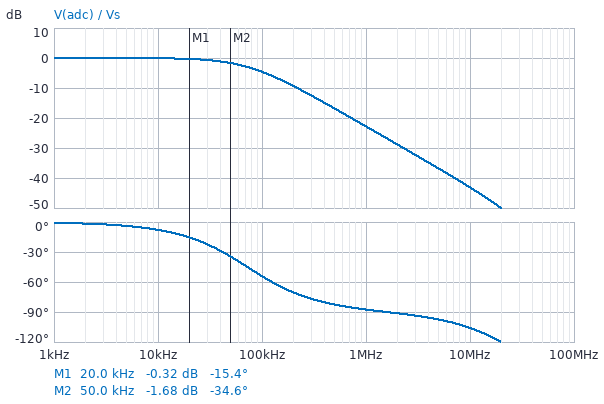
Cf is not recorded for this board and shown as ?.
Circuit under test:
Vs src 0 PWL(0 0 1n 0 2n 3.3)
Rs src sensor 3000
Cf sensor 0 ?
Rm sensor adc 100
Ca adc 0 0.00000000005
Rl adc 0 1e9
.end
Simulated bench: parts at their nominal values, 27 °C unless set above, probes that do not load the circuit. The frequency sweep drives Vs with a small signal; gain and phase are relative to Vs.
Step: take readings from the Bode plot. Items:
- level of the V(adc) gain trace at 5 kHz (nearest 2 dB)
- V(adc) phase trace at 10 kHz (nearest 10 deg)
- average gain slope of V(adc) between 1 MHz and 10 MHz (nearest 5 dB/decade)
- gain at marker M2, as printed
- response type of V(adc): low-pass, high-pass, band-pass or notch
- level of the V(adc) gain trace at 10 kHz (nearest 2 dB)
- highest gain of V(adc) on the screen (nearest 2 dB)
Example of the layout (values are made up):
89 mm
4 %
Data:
0 dB
-10 deg
-20 dB/decade
-1.68 dB
low-pass
0 dB
0 dB
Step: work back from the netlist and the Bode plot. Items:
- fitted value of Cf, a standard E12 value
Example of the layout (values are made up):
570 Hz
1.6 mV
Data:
680 pF
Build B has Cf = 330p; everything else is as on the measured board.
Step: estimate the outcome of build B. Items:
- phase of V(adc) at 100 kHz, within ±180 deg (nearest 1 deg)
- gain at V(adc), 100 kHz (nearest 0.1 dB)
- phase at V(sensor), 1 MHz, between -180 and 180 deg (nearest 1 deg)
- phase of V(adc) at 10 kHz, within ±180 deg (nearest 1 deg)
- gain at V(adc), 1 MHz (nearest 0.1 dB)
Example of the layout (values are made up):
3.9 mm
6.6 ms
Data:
-36 deg
-1.8 dB
-82 deg
-4 deg
-17.2 dB
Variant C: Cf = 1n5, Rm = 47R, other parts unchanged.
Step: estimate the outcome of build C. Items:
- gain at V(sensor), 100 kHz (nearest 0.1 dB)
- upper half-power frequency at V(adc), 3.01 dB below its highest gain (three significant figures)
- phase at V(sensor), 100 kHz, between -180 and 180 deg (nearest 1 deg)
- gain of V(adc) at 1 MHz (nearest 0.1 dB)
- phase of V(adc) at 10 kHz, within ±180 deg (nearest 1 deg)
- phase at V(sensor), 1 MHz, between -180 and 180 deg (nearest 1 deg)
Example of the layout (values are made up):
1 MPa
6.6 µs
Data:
-9.8 dB
34.2 kHz
-71 deg
-29.3 dB
-16 deg
-88 deg
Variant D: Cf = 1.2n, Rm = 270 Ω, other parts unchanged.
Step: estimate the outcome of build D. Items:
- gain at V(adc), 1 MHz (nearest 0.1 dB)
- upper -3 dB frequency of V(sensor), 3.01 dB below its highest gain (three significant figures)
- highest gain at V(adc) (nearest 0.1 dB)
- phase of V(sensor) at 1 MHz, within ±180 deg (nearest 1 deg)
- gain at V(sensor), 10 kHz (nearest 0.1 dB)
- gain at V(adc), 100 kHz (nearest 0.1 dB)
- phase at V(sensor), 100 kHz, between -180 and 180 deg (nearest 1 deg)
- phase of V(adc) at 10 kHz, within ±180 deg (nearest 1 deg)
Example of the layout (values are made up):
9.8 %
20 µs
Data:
-27.5 dB
42.4 kHz
0 dB
-87 deg
-0.2 dB
-8.2 dB
-67 deg
-13 deg
